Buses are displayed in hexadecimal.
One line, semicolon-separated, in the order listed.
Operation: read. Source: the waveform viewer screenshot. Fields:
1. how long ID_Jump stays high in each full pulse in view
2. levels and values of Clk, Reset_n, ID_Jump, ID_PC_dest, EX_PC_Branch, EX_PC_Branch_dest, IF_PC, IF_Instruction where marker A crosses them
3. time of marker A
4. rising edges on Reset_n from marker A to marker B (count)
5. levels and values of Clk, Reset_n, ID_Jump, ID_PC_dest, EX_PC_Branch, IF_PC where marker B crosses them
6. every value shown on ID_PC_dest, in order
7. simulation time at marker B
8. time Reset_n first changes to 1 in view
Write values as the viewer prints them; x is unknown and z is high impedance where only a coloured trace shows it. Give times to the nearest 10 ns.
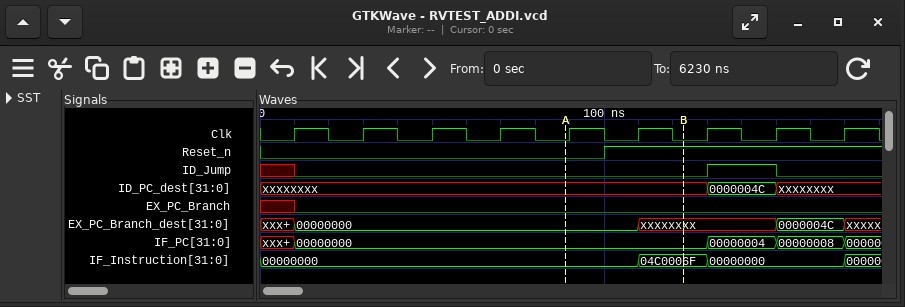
20 ns; Clk=0, Reset_n=0, ID_Jump=0, ID_PC_dest=xxxxxxxx, EX_PC_Branch=0, EX_PC_Branch_dest=00000000, IF_PC=00000000, IF_Instruction=00000000; 90 ns; 1; Clk=0, Reset_n=1, ID_Jump=0, ID_PC_dest=xxxxxxxx, EX_PC_Branch=0, IF_PC=00000000; xxxxxxxx, 0000004C, xxxxxxxx; 120 ns; 100 ns
